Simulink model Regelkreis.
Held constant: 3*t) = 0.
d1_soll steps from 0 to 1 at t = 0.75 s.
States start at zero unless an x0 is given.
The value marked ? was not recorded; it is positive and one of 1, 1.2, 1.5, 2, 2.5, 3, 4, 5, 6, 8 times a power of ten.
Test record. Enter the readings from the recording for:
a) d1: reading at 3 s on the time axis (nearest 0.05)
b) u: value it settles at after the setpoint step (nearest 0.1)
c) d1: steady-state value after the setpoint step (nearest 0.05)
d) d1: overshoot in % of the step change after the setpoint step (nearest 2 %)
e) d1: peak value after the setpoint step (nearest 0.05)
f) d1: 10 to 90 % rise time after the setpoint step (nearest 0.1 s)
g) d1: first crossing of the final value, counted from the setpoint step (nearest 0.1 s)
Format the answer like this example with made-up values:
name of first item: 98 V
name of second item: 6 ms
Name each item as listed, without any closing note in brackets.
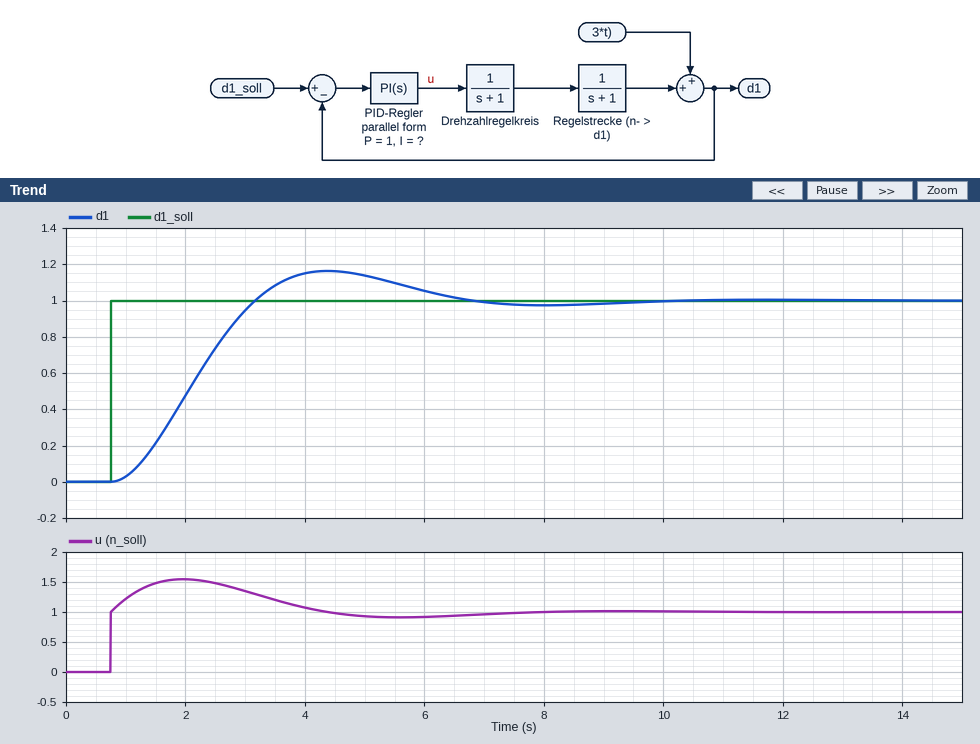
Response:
d1: reading at 3 s on the time axis: 0.95
u: value it settles at after the setpoint step: 1.0
d1: steady-state value after the setpoint step: 1.00
d1: overshoot in % of the step change after the setpoint step: 16 %
d1: peak value after the setpoint step: 1.15
d1: 10 to 90 % rise time after the setpoint step: 1.6 s
d1: first crossing of the final value, counted from the setpoint step: 2.4 s
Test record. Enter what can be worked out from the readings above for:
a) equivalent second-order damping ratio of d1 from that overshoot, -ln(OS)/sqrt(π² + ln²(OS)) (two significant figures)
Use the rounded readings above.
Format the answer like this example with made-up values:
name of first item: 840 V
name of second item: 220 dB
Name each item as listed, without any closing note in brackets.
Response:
equivalent second-order damping ratio of d1 from that overshoot, -ln(OS)/sqrt(π² + ln²(OS)): 0.50
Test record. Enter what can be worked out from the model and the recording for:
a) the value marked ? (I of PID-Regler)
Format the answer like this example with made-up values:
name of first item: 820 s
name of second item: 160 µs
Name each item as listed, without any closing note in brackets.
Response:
the value marked ?: 1
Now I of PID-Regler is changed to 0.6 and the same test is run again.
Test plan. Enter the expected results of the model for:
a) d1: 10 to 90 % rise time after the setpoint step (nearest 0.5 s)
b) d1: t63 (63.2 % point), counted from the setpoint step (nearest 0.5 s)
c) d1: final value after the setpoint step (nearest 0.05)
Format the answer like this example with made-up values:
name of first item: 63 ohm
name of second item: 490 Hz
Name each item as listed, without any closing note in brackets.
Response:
d1: 10 to 90 % rise time after the setpoint step: 2.5 s
d1: t63 (63.2 % point), counted from the setpoint step: 2.0 s
d1: final value after the setpoint step: 1.00
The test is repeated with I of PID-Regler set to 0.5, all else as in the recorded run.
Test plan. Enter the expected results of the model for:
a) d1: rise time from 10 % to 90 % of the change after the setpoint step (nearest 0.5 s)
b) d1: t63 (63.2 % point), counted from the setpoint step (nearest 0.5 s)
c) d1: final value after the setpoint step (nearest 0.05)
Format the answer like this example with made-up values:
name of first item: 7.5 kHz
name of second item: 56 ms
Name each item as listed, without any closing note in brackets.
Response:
d1: rise time from 10 % to 90 % of the change after the setpoint step: 3.0 s
d1: t63 (63.2 % point), counted from the setpoint step: 2.0 s
d1: final value after the setpoint step: 1.00
